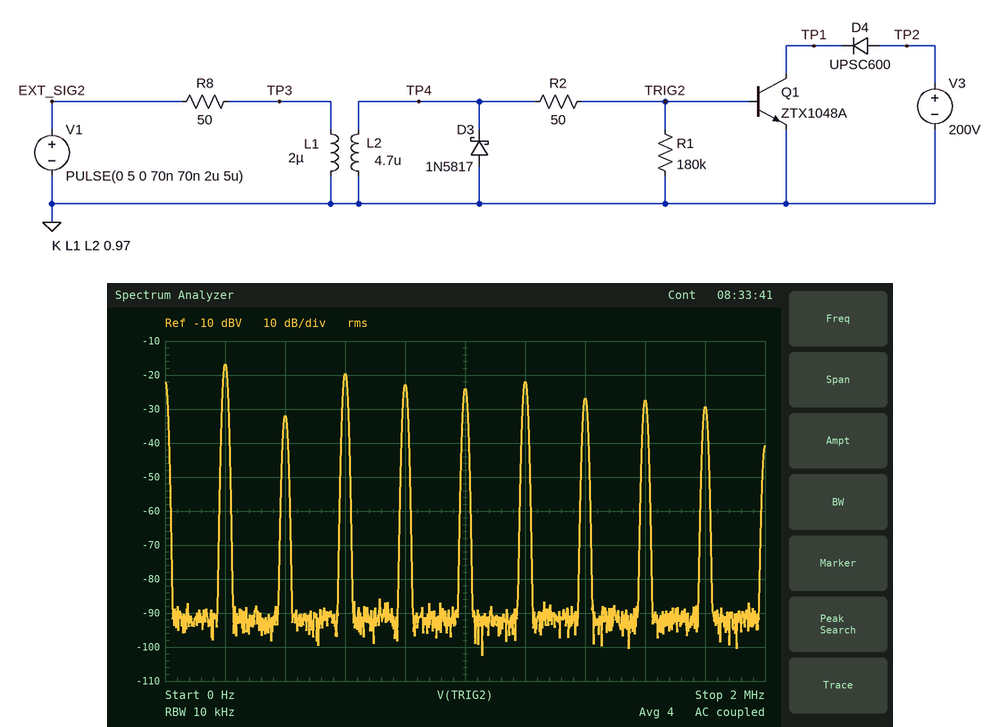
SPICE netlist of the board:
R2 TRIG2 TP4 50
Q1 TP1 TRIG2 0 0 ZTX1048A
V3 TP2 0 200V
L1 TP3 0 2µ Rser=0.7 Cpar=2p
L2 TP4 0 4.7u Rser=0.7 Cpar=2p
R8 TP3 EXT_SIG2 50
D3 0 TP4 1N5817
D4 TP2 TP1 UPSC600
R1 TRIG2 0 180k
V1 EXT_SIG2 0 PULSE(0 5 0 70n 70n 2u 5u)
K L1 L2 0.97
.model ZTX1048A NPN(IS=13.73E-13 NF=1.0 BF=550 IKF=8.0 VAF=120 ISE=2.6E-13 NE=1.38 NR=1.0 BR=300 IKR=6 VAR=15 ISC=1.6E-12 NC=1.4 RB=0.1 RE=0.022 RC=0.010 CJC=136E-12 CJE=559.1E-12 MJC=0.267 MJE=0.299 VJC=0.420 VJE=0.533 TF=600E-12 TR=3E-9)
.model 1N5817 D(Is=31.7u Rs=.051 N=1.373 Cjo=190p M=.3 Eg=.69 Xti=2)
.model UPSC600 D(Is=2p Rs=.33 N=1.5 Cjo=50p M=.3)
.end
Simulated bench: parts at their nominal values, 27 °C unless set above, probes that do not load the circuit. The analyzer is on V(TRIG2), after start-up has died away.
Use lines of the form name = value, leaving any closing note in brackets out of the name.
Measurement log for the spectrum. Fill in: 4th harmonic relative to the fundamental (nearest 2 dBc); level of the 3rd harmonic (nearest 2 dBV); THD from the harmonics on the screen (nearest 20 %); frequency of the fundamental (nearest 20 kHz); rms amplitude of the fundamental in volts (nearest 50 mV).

4th harmonic relative to the fundamental = -6 dBc
level of the 3rd harmonic = -20 dBV
THD from the harmonics on the screen = 120 %
frequency of the fundamental = 200 kHz
rms amplitude of the fundamental in volts = 150 mV
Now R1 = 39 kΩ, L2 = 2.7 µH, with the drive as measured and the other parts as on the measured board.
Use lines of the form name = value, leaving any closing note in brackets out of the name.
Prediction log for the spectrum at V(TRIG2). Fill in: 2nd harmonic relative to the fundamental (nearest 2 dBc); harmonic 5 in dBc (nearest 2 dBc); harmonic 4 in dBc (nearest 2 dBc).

2nd harmonic relative to the fundamental = -14 dBc
harmonic 5 in dBc = -6 dBc
harmonic 4 in dBc = -8 dBc
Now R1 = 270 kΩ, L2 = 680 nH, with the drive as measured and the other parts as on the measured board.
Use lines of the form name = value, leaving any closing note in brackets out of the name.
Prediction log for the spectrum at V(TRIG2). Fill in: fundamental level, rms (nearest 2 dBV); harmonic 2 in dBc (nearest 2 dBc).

fundamental level, rms = -24 dBV
harmonic 2 in dBc = -8 dBc
